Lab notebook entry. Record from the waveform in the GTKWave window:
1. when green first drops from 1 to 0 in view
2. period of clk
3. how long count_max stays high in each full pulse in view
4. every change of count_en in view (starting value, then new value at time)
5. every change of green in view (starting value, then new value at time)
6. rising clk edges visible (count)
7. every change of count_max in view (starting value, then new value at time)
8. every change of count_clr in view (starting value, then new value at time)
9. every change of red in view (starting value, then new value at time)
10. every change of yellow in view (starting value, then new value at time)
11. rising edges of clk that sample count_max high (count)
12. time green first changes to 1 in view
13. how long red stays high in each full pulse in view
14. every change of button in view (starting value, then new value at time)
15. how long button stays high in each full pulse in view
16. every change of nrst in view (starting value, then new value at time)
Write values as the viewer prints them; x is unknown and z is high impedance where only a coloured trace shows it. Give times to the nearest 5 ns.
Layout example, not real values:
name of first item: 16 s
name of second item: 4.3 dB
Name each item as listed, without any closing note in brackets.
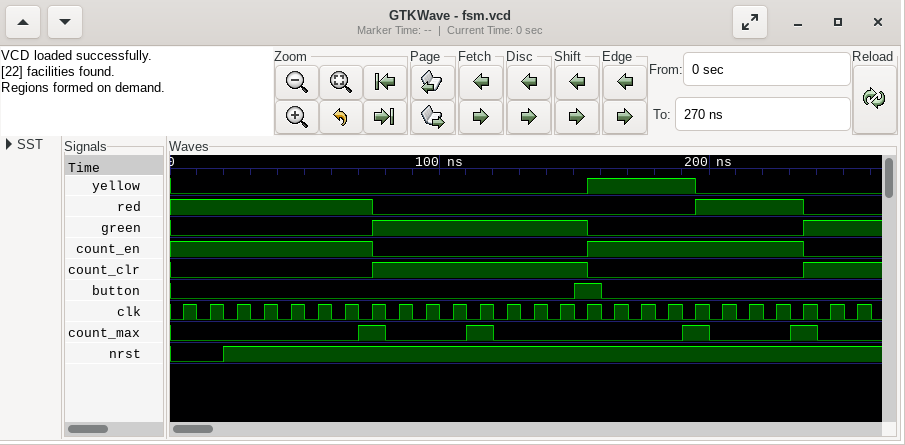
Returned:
when green first drops from 1 to 0 in view: 155 ns
period of clk: 10 ns
how long count_max stays high in each full pulse in view: 10 ns, 10 ns, 10 ns, 10 ns
every change of count_en in view: 1, 0 at 75 ns, 1 at 155 ns, 0 at 235 ns
every change of green in view: 0, 1 at 75 ns, 0 at 155 ns, 1 at 235 ns
rising clk edges visible: 26
every change of count_max in view: 0, 1 at 70 ns, 0 at 80 ns, 1 at 110 ns, 0 at 120 ns, 1 at 190 ns, 0 at 200 ns, 1 at 230 ns, 0 at 240 ns
every change of count_clr in view: 0, 1 at 75 ns, 0 at 155 ns, 1 at 235 ns
every change of red in view: 1, 0 at 75 ns, 1 at 195 ns, 0 at 235 ns
every change of yellow in view: 0, 1 at 155 ns, 0 at 195 ns
rising edges of clk that sample count_max high: 4
time green first changes to 1 in view: 75 ns
how long red stays high in each full pulse in view: 40 ns
every change of button in view: 0, 1 at 150 ns, 0 at 160 ns
how long button stays high in each full pulse in view: 10 ns
every change of nrst in view: 0, 1 at 20 ns
